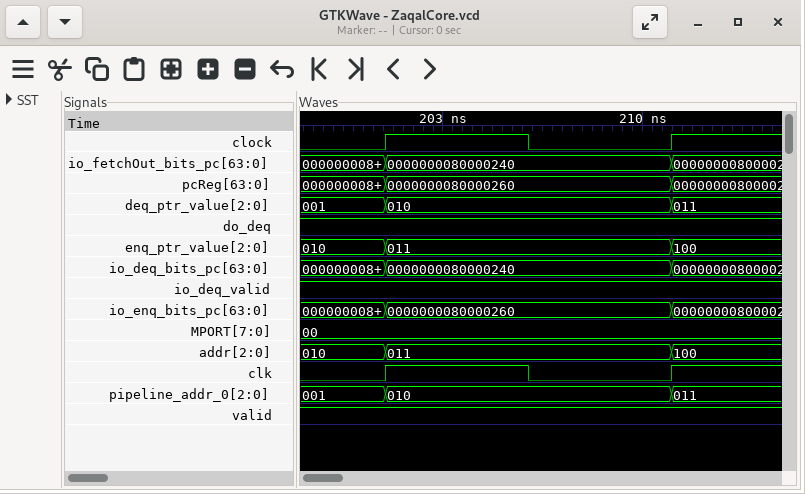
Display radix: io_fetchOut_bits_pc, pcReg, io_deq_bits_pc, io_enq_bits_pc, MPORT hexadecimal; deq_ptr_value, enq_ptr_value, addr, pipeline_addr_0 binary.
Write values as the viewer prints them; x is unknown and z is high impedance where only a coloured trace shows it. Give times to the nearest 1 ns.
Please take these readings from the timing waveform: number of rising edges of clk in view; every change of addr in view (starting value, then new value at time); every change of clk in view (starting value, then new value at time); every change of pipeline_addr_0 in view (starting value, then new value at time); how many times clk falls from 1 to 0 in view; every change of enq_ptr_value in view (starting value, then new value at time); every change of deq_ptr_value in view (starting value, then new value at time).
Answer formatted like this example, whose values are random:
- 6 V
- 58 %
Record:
- 2
- 010, 011 at 201 ns, 100 at 211 ns
- 0, 1 at 201 ns, 0 at 206 ns, 1 at 211 ns
- 001, 010 at 201 ns, 011 at 211 ns
- 1
- 010, 011 at 201 ns, 100 at 211 ns
- 001, 010 at 201 ns, 011 at 211 ns
